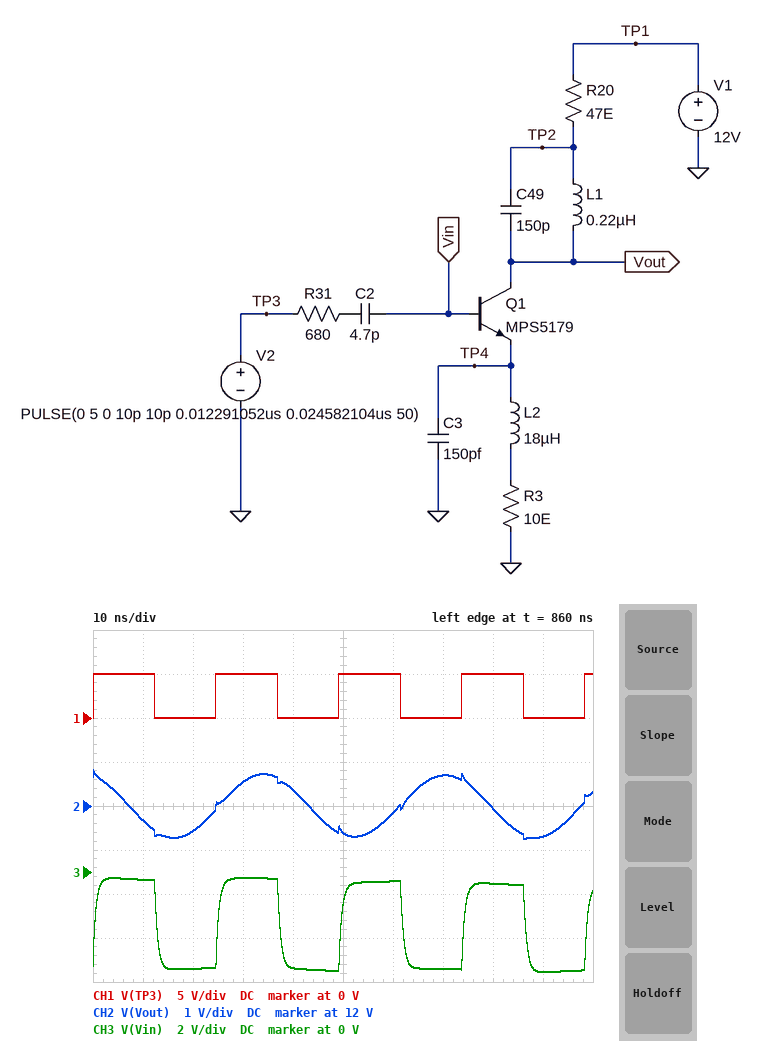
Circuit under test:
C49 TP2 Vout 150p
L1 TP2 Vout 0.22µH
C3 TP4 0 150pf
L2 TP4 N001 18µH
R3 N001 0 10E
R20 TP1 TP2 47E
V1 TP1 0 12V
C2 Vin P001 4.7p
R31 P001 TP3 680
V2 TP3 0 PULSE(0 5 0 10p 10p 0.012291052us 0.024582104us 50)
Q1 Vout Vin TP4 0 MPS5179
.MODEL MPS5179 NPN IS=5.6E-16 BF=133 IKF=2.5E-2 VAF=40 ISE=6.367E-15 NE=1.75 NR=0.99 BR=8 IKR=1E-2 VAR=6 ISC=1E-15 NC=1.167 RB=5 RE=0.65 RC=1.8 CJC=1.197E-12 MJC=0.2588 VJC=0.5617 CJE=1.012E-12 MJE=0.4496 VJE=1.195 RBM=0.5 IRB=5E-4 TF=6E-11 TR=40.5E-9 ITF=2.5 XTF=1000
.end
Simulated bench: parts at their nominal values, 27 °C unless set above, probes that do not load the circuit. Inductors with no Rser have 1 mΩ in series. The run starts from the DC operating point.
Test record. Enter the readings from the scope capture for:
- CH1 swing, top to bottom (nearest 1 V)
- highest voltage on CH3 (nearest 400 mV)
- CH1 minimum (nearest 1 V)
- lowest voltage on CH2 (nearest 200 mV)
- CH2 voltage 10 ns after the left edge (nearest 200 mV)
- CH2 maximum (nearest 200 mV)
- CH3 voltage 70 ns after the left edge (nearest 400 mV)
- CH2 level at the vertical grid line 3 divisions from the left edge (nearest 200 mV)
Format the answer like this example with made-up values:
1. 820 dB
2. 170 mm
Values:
1. 5 V
2. -400 mV
3. 0 V
4. 11.2 V
5. 11.6 V
6. 12.8 V
7. -4.4 V
8. 12.6 V
